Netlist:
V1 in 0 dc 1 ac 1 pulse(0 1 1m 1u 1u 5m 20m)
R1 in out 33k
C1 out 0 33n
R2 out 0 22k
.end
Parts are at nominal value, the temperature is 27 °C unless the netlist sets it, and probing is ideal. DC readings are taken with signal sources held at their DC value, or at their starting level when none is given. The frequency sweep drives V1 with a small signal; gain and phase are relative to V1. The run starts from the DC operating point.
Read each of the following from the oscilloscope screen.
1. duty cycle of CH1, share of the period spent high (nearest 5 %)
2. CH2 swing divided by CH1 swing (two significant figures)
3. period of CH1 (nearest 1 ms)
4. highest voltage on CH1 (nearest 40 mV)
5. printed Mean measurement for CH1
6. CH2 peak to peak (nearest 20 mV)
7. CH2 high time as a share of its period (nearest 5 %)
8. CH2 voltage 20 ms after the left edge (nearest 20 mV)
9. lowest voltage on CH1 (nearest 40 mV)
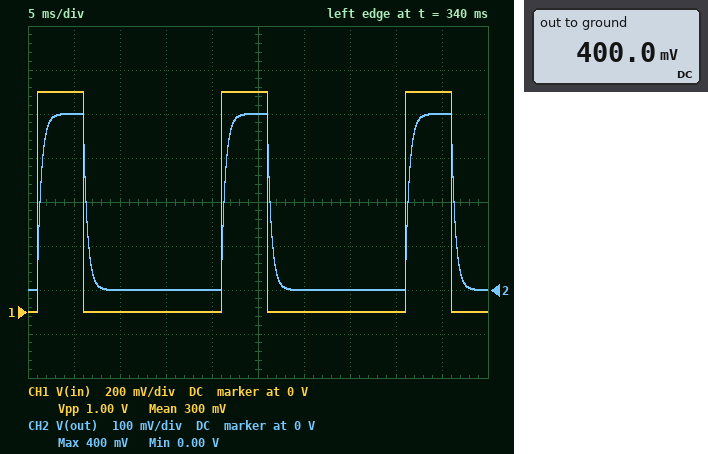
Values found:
25 %
0.40
20 ms
1.00 V
300 mV
400 mV
25 %
0 V
0 V
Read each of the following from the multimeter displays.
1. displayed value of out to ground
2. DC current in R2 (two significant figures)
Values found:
400.0 mV
18 µA
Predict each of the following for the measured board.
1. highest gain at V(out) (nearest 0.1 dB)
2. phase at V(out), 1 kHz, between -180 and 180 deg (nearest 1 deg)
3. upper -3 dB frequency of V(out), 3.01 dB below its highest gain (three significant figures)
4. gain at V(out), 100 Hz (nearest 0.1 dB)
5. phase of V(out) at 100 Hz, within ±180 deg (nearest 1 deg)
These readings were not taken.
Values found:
-8.0 dB
-70 deg
365 Hz
-8.3 dB
-15 deg
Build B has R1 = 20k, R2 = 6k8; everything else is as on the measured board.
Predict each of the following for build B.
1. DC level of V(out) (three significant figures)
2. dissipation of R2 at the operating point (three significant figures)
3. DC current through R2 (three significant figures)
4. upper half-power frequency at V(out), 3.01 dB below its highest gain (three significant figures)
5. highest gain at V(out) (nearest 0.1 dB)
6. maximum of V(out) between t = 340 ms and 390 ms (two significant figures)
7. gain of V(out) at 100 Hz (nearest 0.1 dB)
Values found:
254 mV
9.47 µW
37.3 µA
950 Hz
-11.9 dB
250 mV
-12.0 dB
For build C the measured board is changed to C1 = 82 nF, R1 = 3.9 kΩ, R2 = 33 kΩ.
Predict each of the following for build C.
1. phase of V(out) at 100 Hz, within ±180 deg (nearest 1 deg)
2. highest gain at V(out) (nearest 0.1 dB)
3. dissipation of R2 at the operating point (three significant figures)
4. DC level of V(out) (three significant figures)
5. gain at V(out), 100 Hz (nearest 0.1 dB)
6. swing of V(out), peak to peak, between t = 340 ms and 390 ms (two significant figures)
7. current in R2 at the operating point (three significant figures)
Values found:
-10 deg
-1.0 dB
24.2 µW
894 mV
-1.1 dB
890 mV
27.1 µA
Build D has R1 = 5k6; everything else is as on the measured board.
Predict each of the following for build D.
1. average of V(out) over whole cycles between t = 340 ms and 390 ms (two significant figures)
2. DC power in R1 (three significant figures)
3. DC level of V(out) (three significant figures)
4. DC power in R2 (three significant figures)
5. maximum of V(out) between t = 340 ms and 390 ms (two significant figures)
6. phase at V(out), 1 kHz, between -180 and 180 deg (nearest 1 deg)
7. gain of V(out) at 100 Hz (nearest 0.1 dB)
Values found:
200 mV
7.35 µW
797 mV
28.9 µW
800 mV
-43 deg
-2.0 dB
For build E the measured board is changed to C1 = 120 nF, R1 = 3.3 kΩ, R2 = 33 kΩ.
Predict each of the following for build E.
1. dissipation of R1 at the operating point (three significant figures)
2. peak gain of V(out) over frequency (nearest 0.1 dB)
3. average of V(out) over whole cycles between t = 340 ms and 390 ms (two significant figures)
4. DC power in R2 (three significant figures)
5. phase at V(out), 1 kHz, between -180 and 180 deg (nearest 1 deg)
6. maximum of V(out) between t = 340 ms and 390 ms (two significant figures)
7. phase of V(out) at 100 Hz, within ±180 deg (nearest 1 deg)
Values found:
2.50 µW
-0.8 dB
230 mV
25.0 µW
-66 deg
910 mV
-13 deg
